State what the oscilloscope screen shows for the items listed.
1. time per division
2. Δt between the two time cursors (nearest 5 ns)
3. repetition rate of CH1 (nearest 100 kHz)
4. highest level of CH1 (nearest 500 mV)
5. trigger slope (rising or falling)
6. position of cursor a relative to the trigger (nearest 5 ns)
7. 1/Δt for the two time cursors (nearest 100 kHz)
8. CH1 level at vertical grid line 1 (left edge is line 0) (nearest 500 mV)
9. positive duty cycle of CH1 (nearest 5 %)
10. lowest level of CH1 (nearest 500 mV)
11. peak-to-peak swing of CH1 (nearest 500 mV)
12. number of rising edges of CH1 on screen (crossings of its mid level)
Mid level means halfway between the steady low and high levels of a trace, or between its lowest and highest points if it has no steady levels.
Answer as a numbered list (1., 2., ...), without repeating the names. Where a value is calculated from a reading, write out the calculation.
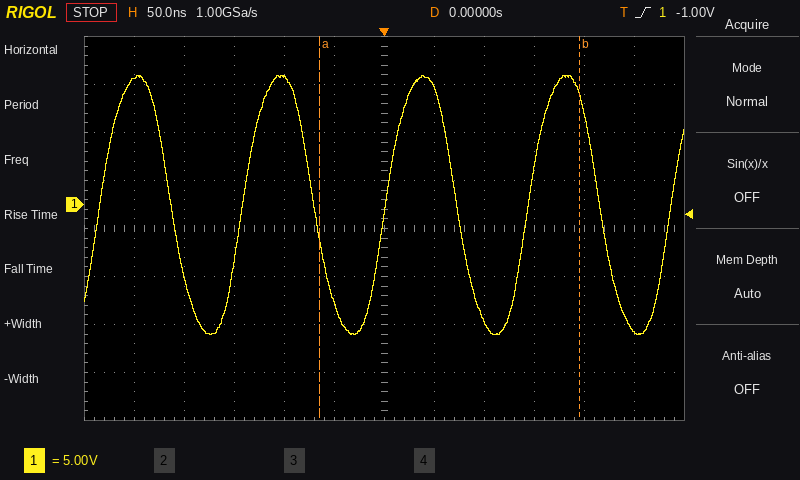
1. 50 ns
2. 260 ns
3. 7.0 MHz
4. 13.5 V
5. rising
6. -65 ns
7. 1 / 260 ns ≈ 3.8 MHz
8. 13.0 V
9. 50 %
10. -13.5 V
11. 13.5 V − (-13.5 V) = 27.0 V
12. 5
